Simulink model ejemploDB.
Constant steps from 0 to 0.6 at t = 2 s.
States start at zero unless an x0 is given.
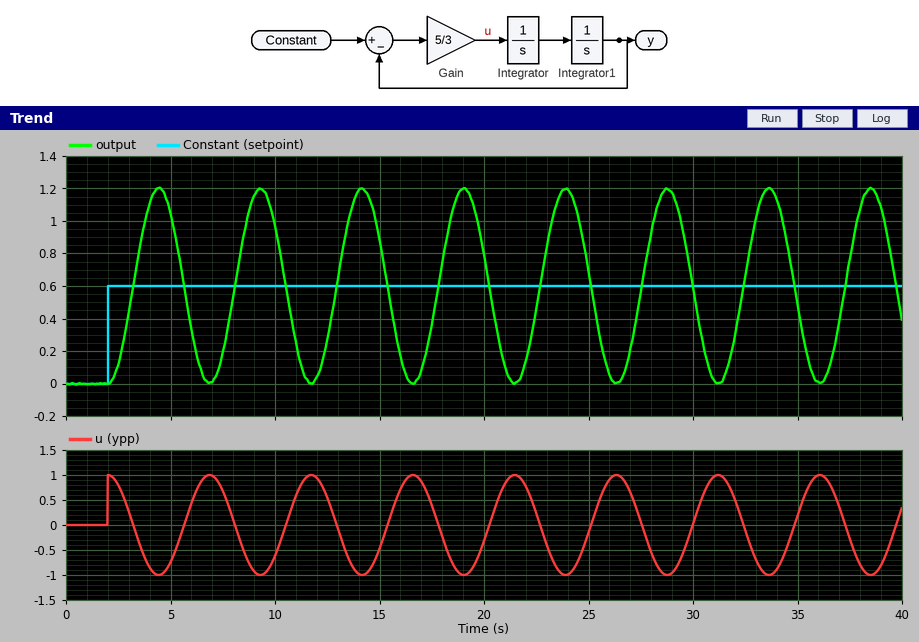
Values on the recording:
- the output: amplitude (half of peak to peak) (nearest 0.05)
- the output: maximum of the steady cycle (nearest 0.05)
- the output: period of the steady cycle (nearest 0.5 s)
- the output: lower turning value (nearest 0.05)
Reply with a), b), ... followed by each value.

a) 0.60
b) 1.20
c) 5.0 s
d) 0.00
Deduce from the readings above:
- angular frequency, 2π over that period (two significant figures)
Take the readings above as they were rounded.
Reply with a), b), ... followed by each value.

a) 1.3 rad/s
